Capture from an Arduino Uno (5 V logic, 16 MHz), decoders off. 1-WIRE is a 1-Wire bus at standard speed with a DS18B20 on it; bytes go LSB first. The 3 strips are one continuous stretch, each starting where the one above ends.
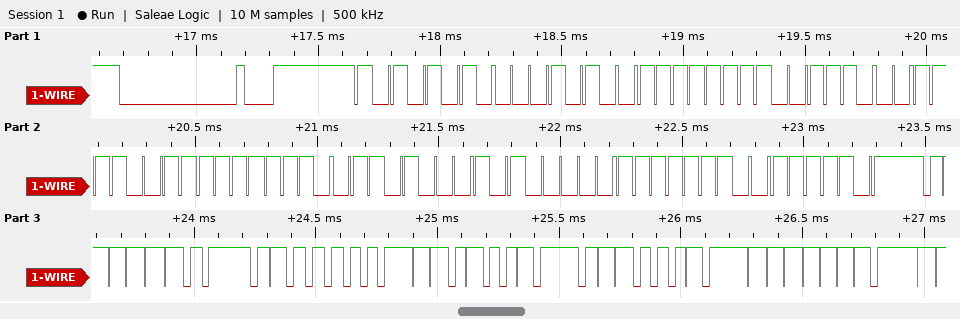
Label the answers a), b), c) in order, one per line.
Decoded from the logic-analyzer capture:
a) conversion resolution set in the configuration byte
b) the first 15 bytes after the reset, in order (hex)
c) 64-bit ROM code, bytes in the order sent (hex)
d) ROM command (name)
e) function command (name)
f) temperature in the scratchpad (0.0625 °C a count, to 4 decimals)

a) 12 bits
b) 55 28 FF 1C CF 7F 16 05 7F BE 3E 02 4B 46 7F
c) 28 FF 1C CF 7F 16 05 7F
d) Match ROM
e) Read Scratchpad
f) 35.8750 °C
